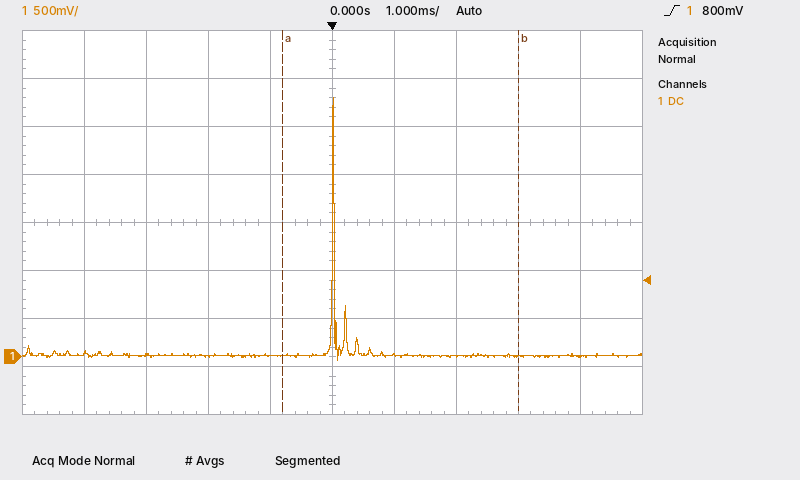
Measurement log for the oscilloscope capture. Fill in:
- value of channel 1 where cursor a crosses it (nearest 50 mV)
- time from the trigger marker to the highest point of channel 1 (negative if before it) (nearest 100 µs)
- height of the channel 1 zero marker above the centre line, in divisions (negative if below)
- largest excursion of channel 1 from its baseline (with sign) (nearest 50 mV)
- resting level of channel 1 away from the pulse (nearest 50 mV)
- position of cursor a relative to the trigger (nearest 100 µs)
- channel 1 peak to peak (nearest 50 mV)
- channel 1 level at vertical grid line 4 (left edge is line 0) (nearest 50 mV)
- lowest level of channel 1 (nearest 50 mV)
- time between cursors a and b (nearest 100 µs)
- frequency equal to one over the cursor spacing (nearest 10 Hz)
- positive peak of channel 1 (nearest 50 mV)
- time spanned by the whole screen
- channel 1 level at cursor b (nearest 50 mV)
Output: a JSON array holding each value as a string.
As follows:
["0 mV", "0.0 ms", "-2.8 div", "+2.70 V", "0 mV", "-800 µs", "2.75 V", "0 mV", "-50 mV", "3.8 ms", "260 Hz", "2.70 V", "10 ms", "0 mV"]
